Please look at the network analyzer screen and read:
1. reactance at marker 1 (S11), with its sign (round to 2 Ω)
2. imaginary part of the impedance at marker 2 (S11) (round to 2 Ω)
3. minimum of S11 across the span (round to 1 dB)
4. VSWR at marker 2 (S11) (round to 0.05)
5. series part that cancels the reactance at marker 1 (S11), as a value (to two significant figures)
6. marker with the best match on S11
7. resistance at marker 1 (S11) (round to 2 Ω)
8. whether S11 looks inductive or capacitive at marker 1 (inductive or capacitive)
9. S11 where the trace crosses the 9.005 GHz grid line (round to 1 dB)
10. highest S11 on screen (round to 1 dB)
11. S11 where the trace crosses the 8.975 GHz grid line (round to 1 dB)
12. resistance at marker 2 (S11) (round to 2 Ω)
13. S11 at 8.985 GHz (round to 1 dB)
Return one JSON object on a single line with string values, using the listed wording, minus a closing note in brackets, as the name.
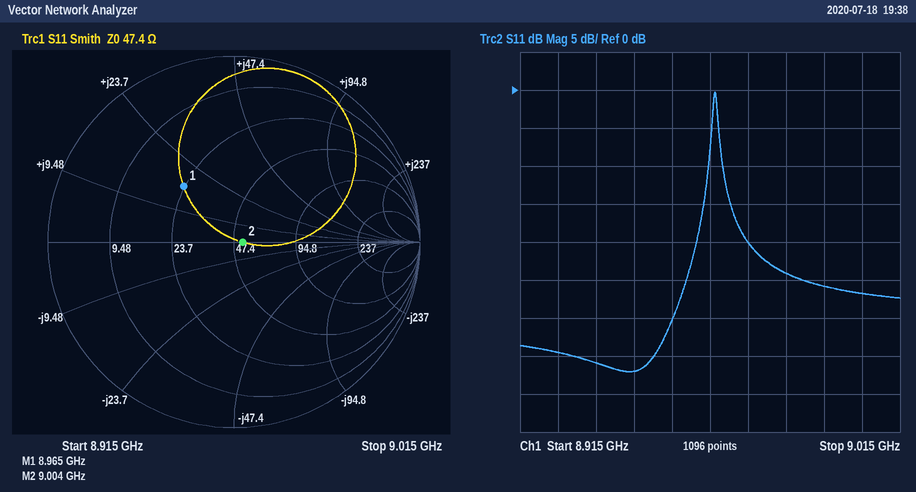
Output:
{"reactance at marker 1 (S11), with its sign": "+16 Ω", "imaginary part of the impedance at marker 2 (S11)": "0 Ω", "minimum of S11 across the span": "-37 dB", "VSWR at marker 2 (S11)": "1.10", "series part that cancels the reactance at marker 1 (S11), as a value": "1.1 pF", "marker with the best match on S11": "marker 2", "resistance at marker 1 (S11)": "24 Ω", "whether S11 looks inductive or capacitive at marker 1": "inductive", "S11 where the trace crosses the 9.005 GHz grid line": "-27 dB", "highest S11 on screen": "0 dB", "S11 where the trace crosses the 8.975 GHz grid line": "-20 dB", "resistance at marker 2 (S11)": "52 Ω", "S11 at 8.985 GHz": "-24 dB"}
